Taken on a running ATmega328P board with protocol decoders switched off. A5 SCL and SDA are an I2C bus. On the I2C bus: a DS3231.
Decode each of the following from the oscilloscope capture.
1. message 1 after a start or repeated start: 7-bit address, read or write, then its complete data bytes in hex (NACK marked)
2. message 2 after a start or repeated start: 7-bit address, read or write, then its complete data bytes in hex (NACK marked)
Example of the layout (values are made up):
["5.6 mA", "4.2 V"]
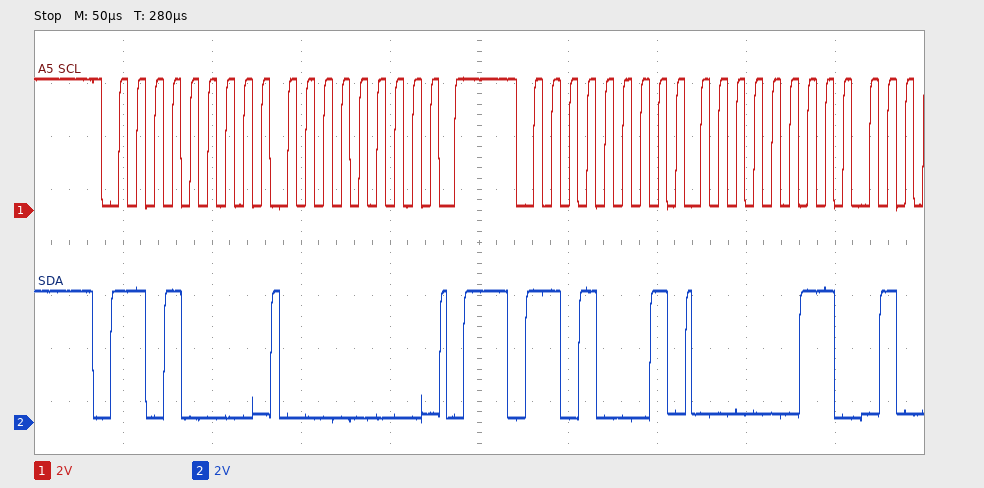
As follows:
["0x68 write: 00", "0x68 read: 03"]
